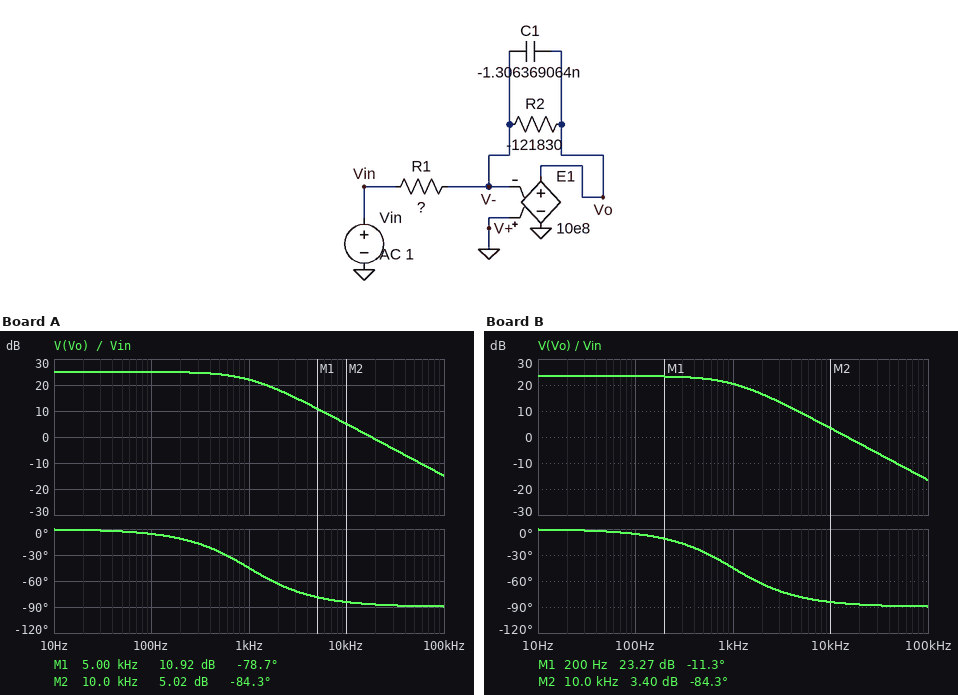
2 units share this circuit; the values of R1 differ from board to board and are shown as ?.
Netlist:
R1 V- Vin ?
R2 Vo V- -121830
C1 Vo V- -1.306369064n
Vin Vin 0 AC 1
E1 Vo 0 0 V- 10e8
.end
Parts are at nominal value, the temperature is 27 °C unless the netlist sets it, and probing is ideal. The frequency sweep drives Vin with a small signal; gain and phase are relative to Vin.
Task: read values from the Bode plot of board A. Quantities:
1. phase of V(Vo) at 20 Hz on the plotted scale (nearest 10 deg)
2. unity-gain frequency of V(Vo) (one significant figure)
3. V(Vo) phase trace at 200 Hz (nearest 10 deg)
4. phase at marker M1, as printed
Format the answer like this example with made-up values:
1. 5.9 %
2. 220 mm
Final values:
1. 0 deg
2. 20 kHz
3. -10 deg
4. -78.7 deg
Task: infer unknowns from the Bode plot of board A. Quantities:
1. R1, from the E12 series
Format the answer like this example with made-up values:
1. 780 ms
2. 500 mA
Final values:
1. 6.8 kΩ
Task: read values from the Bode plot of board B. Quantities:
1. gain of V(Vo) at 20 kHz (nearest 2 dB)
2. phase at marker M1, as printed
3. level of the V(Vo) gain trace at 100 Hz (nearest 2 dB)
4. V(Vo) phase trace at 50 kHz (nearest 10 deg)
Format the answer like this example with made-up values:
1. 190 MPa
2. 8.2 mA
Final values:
1. -2 dB
2. -11.3 deg
3. 24 dB
4. -90 deg
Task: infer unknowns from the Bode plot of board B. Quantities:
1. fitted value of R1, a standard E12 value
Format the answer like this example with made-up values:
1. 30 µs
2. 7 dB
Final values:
1. 8.2 kΩ
